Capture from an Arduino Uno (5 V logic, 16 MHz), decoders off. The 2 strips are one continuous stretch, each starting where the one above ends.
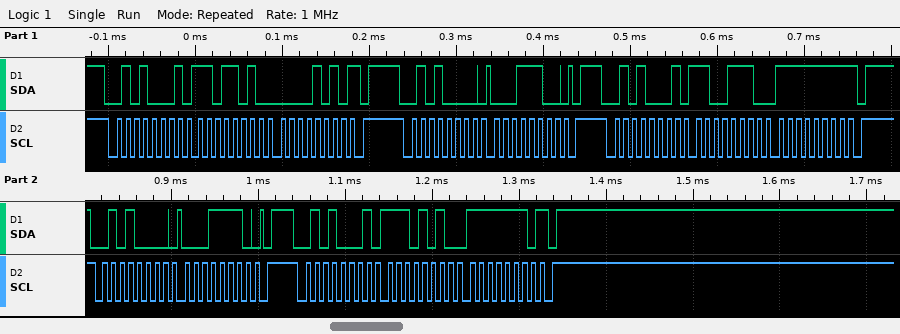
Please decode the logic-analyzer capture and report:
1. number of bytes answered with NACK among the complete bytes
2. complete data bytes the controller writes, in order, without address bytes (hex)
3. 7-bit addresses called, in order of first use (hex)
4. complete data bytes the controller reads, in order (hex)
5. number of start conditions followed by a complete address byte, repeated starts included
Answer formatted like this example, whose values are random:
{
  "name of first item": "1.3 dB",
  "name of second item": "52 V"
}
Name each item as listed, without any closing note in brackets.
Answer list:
{
  "number of bytes answered with NACK among the complete bytes": "3",
  "complete data bytes the controller writes, in order, without address bytes": "1C 1E",
  "7-bit addresses called, in order of first use": "0x28",
  "complete data bytes the controller reads, in order": "DA 0A CE FF EA FE",
  "number of start conditions followed by a complete address byte, repeated starts included": "5"
}
